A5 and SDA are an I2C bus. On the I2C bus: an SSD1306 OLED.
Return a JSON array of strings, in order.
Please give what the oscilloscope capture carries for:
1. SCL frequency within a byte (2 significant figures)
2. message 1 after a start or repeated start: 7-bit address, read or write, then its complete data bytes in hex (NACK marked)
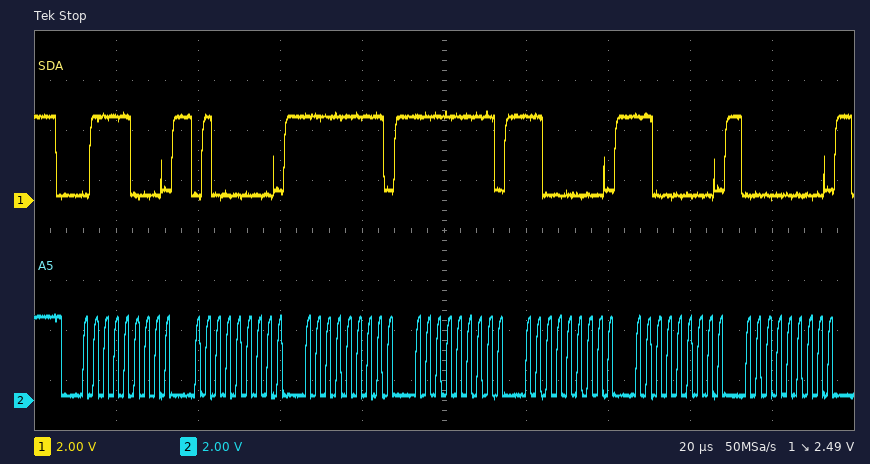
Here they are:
["400 kHz", "0x3C write: 40 FF FF C0 C0 00"]
